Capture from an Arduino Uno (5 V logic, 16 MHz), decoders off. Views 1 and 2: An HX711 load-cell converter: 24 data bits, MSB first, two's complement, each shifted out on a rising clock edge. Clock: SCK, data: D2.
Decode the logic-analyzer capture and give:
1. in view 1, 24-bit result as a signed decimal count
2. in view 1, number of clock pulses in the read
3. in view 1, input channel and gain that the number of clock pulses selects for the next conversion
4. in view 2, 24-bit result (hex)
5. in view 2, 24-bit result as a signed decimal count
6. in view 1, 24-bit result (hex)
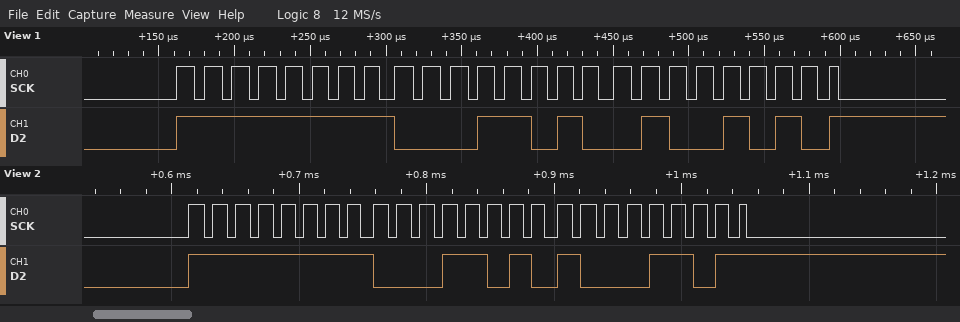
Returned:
-58806
25
channel A, gain 128
0xFF1A8D
-58739
0xFF1A4A
